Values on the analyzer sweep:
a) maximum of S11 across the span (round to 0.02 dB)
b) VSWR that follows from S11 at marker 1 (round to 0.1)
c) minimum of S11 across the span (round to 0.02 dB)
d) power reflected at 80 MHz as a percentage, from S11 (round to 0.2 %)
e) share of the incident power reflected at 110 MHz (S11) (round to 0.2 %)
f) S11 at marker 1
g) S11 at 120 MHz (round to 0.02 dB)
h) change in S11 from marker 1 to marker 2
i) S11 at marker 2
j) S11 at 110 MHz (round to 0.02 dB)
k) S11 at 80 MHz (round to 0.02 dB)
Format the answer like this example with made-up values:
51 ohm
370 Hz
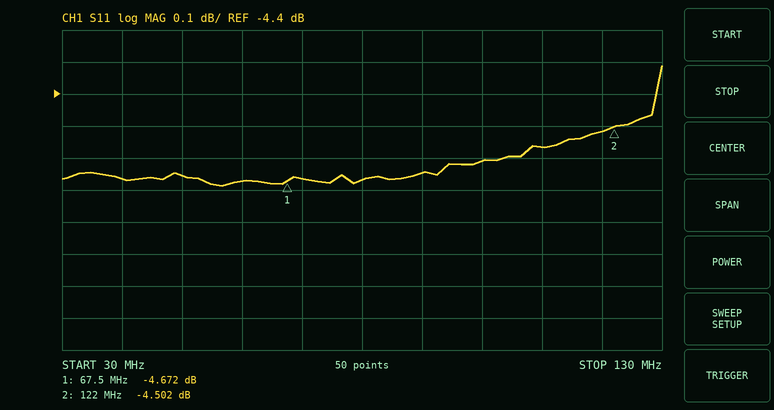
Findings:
-4.32 dB
3.8
-4.68 dB
34.2 %
35.0 %
-4.672 dB
-4.52 dB
0.170 dB
-4.502 dB
-4.56 dB
-4.66 dB
